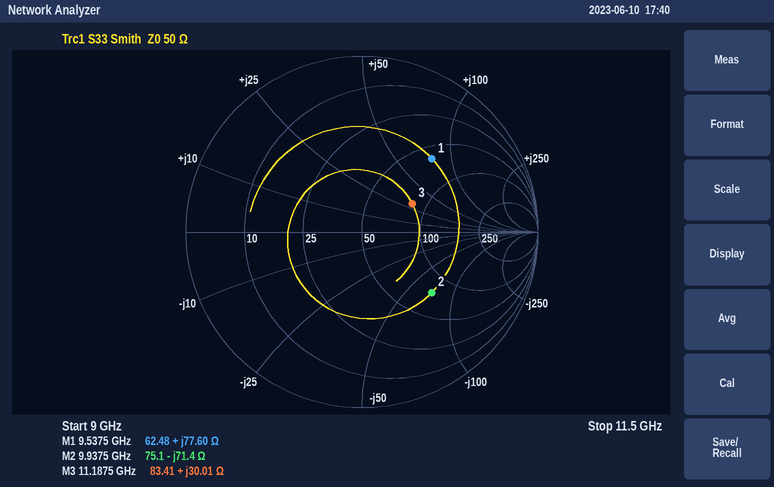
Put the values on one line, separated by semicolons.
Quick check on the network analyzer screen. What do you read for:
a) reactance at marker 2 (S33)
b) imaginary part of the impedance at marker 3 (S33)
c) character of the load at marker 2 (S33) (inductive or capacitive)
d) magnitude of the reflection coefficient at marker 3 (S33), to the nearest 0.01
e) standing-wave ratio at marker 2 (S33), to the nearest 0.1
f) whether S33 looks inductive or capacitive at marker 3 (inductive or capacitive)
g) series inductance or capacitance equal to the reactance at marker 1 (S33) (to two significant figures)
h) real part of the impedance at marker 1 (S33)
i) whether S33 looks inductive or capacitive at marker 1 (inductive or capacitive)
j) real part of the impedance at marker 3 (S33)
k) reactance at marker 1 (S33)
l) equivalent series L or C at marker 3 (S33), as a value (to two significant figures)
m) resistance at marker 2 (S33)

-71.4 Ω; +30.01 Ω; capacitive; 0.33; 3.2; inductive; 1.3 nH; 62.48 Ω; inductive; 83.41 Ω; +77.60 Ω; 430 pH; 75.1 Ω
